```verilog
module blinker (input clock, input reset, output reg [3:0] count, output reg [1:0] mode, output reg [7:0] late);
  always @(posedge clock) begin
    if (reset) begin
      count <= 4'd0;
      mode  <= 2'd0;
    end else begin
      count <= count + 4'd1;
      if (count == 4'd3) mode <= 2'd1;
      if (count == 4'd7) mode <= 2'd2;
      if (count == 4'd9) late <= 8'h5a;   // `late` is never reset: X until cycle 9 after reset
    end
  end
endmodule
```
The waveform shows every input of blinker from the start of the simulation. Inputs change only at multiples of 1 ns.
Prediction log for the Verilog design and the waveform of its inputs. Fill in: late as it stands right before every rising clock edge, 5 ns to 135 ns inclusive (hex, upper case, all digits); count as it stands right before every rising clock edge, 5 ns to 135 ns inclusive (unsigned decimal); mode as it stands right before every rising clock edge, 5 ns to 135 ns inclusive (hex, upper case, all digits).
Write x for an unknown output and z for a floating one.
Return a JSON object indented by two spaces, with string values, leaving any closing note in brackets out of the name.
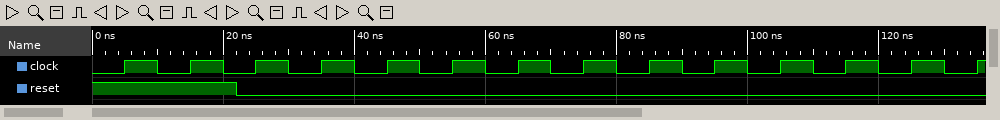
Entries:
{
  "late as it stands right before every rising clock edge, 5 ns to 135 ns inclusive": "x, x, x, x, x, x, x, x, x, x, x, x, 5A, 5A",
  "count as it stands right before every rising clock edge, 5 ns to 135 ns inclusive": "x, 0, 0, 1, 2, 3, 4, 5, 6, 7, 8, 9, 10, 11",
  "mode as it stands right before every rising clock edge, 5 ns to 135 ns inclusive": "x, 0, 0, 0, 0, 0, 1, 1, 1, 1, 2, 2, 2, 2"
}
